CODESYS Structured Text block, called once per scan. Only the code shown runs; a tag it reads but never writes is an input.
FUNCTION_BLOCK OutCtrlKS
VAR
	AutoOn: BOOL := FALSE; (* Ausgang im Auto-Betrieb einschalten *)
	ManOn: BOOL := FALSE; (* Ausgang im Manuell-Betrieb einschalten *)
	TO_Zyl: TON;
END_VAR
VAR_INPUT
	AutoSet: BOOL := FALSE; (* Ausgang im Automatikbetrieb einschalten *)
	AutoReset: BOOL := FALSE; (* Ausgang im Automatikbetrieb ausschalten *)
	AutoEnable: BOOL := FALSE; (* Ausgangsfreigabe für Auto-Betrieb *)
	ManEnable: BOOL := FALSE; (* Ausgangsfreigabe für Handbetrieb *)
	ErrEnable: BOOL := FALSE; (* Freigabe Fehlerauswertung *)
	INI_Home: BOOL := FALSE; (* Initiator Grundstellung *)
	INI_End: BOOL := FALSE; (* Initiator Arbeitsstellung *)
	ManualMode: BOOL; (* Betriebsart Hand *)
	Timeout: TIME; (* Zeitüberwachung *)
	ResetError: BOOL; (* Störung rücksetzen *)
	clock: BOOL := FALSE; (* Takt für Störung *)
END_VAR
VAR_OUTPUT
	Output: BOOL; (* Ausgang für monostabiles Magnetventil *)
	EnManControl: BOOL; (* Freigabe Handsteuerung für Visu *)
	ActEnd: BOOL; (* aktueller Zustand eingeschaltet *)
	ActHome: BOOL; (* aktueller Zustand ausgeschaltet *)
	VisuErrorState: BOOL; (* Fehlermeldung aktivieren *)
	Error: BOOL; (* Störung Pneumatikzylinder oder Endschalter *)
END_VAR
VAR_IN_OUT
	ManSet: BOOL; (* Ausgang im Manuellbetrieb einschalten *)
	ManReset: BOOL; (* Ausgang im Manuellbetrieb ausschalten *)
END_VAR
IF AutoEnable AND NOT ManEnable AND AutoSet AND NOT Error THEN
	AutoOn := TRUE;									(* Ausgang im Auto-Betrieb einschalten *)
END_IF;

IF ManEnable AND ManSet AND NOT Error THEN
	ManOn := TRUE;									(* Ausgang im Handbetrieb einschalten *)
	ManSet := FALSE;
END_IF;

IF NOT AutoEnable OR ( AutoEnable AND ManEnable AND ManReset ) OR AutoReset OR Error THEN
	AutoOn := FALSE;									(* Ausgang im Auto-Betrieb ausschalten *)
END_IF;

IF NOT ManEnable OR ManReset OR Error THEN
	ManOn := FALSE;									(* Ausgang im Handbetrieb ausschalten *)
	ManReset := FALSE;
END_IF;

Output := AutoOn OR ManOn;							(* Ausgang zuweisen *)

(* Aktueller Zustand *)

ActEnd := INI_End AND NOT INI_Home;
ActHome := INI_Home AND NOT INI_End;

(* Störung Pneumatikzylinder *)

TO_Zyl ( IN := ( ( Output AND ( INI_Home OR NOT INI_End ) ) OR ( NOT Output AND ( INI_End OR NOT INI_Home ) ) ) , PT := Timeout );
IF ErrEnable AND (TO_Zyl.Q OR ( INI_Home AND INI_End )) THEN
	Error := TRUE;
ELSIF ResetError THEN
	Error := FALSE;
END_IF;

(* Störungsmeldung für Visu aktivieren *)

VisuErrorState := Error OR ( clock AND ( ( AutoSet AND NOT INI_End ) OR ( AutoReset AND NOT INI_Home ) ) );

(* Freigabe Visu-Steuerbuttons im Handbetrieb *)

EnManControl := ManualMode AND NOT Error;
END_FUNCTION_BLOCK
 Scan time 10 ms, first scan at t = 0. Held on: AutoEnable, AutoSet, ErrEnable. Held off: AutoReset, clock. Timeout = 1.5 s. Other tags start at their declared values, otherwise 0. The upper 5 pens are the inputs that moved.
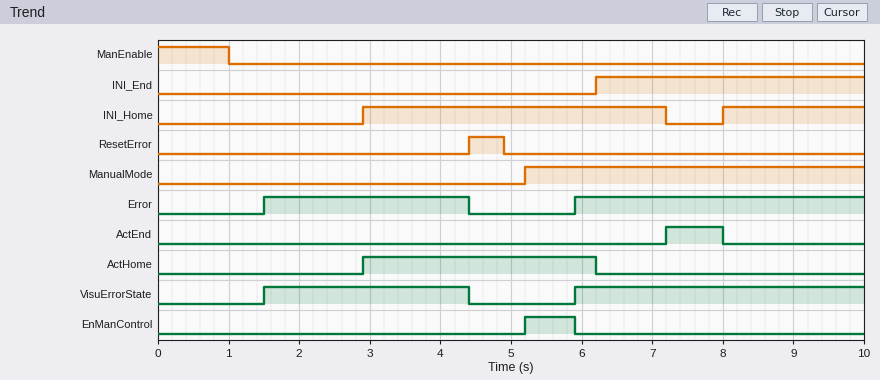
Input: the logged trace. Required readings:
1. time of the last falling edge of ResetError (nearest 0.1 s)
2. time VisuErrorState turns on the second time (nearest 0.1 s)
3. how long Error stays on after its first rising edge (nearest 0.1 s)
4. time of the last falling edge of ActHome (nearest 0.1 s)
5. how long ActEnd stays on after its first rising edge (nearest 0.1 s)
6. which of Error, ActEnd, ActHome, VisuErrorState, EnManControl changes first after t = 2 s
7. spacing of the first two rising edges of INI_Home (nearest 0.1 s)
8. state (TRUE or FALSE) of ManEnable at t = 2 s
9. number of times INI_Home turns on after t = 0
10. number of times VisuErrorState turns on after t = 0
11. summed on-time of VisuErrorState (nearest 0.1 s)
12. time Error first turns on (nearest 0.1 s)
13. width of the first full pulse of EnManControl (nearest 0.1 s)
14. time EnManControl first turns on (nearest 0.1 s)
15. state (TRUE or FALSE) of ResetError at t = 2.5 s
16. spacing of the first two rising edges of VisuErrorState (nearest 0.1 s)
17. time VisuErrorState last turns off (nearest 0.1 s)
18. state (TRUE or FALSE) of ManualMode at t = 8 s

4.9 s
5.9 s
2.9 s
6.2 s
0.8 s
ActHome
5.1 s
FALSE
2
2
7.0 s
1.5 s
0.7 s
5.2 s
FALSE
4.4 s
4.4 s
TRUE
